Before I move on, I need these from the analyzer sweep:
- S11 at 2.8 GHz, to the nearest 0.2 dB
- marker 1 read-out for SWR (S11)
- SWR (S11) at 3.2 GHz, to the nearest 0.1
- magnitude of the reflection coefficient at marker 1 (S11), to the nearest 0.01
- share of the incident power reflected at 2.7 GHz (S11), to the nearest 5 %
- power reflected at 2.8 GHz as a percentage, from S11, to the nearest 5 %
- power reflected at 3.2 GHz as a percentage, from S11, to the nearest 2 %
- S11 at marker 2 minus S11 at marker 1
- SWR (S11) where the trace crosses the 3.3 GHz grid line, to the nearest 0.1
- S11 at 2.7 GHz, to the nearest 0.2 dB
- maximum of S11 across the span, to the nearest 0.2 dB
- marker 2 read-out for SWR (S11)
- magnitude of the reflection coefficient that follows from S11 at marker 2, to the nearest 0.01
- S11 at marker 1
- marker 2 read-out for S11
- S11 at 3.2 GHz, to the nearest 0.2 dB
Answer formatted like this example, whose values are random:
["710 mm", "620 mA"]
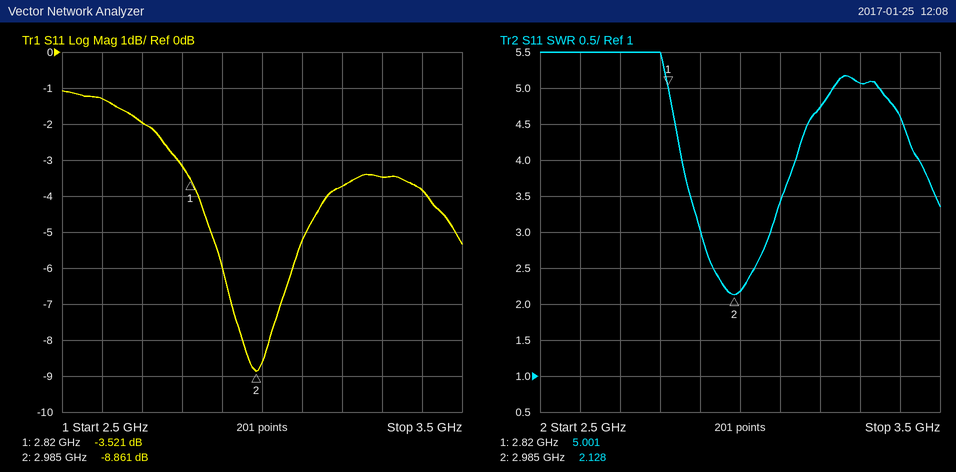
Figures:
["-3.2 dB", "5.001", "4.7", "0.67", "65 %", "50 %", "42 %", "-5.340 dB", "5.1", "-2.0 dB", "-1.0 dB", "2.128", "0.36", "-3.521 dB", "-8.861 dB", "-3.8 dB"]
